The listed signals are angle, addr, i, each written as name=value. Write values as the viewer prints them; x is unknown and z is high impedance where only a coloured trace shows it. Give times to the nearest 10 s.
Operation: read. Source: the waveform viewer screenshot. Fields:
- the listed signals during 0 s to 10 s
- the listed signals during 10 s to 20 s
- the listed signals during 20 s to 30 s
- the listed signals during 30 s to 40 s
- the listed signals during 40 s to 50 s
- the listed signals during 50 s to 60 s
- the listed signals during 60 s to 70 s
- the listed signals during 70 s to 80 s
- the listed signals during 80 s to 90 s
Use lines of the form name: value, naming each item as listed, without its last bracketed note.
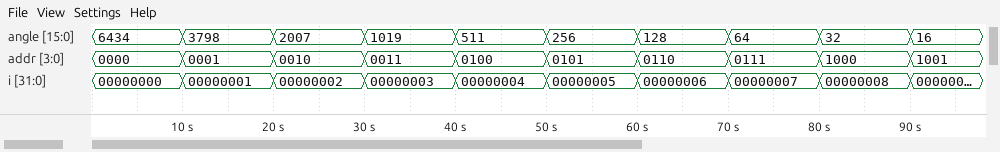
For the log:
the listed signals during 0 s to 10 s: angle=6434, addr=0000, i=00000000
the listed signals during 10 s to 20 s: angle=3798, addr=0001, i=00000001
the listed signals during 20 s to 30 s: angle=2007, addr=0010, i=00000002
the listed signals during 30 s to 40 s: angle=1019, addr=0011, i=00000003
the listed signals during 40 s to 50 s: angle=511, addr=0100, i=00000004
the listed signals during 50 s to 60 s: angle=256, addr=0101, i=00000005
the listed signals during 60 s to 70 s: angle=128, addr=0110, i=00000006
the listed signals during 70 s to 80 s: angle=64, addr=0111, i=00000007
the listed signals during 80 s to 90 s: angle=32, addr=1000, i=00000008
